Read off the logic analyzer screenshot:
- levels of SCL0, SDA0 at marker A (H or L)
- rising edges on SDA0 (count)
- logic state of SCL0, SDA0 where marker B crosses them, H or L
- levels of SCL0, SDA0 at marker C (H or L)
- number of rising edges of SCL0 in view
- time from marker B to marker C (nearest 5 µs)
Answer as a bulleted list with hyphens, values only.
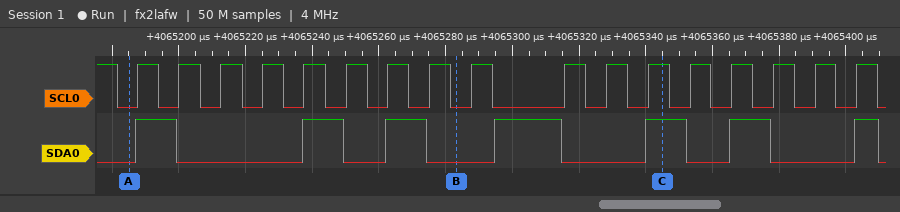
- SCL0=L, SDA0=L
- 7
- SCL0=L, SDA0=L
- SCL0=H, SDA0=H
- 17
- 60 µs
